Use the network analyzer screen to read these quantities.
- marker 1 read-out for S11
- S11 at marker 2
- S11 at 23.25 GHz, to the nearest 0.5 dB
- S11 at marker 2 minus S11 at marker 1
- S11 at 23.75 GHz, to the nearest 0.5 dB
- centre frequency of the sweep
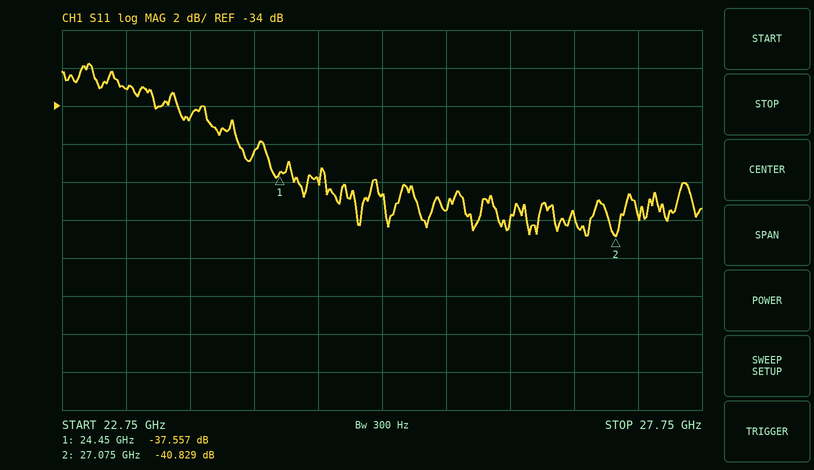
-37.557 dB
-40.829 dB
-33.0 dB
-3.272 dB
-34.5 dB
25.25 GHz
